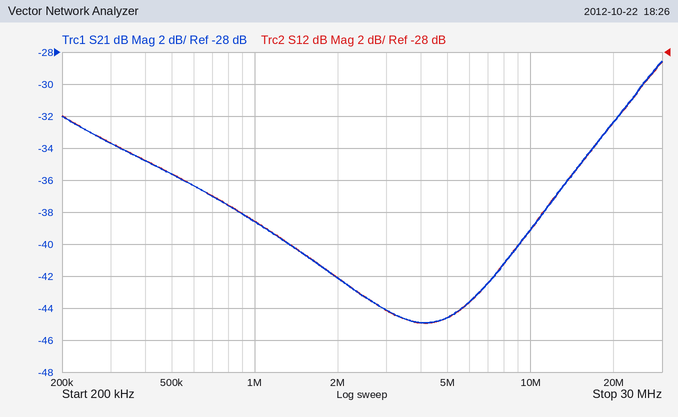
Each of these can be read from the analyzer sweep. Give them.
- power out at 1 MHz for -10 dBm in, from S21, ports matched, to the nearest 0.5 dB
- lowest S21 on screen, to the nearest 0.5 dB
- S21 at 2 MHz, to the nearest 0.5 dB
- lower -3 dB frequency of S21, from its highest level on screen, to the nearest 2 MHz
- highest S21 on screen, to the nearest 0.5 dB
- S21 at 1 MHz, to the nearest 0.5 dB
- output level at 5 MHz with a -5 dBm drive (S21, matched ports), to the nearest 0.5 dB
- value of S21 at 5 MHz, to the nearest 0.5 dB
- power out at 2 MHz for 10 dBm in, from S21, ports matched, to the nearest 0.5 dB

-48.5 dBm
-45.0 dB
-42.0 dB
22 MHz
-28.5 dB
-38.5 dB
-49.5 dBm
-44.5 dB
-32.0 dBm
